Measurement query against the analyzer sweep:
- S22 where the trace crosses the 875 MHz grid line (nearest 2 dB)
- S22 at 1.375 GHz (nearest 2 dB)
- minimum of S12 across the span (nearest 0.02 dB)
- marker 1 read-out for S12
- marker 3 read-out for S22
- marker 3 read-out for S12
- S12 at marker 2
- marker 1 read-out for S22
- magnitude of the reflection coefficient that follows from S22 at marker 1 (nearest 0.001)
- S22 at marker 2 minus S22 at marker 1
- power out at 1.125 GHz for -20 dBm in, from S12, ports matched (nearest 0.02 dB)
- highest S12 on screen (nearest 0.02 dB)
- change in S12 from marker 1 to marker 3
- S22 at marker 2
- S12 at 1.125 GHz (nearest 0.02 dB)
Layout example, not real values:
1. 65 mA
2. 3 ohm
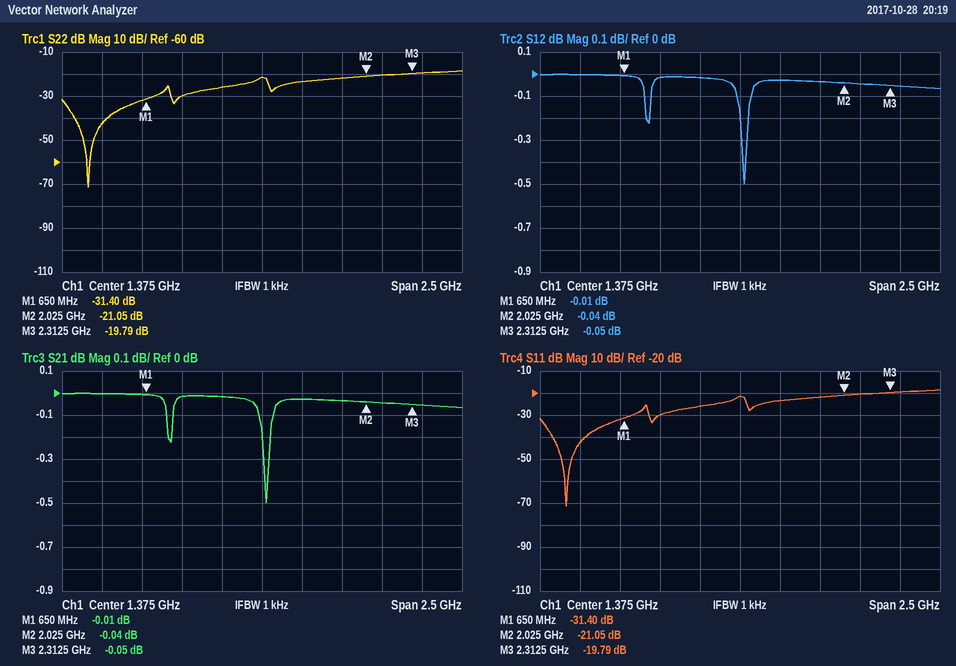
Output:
1. -30 dB
2. -22 dB
3. -0.50 dB
4. -0.01 dB
5. -19.79 dB
6. -0.05 dB
7. -0.04 dB
8. -31.40 dB
9. 0.027
10. 10.35 dB
11. -20.02 dBm
12. 0.00 dB
13. -0.04 dB
14. -21.05 dB
15. -0.02 dB
